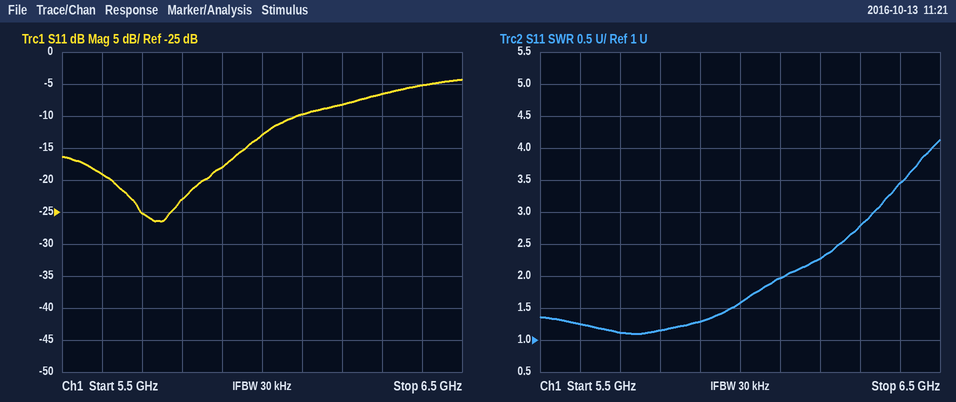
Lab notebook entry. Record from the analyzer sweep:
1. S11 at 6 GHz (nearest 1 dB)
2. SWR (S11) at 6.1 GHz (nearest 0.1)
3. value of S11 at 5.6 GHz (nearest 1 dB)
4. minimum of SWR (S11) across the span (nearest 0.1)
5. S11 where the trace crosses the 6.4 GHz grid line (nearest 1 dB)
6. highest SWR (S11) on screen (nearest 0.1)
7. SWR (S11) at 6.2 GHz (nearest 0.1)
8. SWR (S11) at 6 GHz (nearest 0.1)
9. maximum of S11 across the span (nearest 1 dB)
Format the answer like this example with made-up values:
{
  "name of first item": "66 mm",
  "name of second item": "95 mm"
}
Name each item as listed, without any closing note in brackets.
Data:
{
  "S11 at 6 GHz": "-13 dB",
  "SWR (S11) at 6.1 GHz": "2.0",
  "value of S11 at 5.6 GHz": "-19 dB",
  "minimum of SWR (S11) across the span": "1.1",
  "S11 where the trace crosses the 6.4 GHz grid line": "-5 dB",
  "highest SWR (S11) on screen": "4.1",
  "SWR (S11) at 6.2 GHz": "2.3",
  "SWR (S11) at 6 GHz": "1.6",
  "maximum of S11 across the span": "-4 dB"
}
